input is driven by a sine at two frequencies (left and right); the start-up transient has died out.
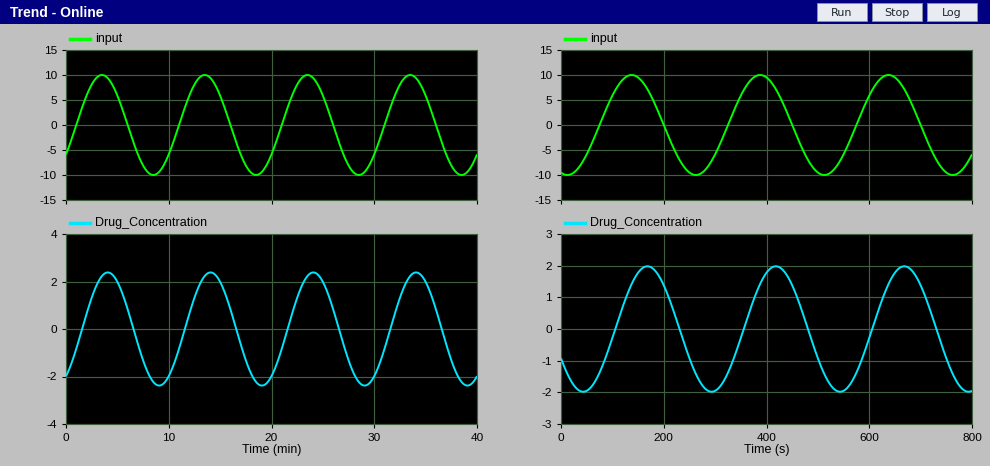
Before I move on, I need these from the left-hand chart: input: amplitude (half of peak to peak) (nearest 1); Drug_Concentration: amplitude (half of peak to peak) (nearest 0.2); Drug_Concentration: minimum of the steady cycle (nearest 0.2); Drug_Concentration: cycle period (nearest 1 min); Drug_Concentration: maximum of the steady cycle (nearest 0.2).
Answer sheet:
10
2.4
-2.4
10 min
2.4
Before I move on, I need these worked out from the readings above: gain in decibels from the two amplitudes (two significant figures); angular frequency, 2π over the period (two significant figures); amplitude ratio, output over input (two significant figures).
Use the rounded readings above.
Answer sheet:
-12 dB
0.63 rad/min
0.24
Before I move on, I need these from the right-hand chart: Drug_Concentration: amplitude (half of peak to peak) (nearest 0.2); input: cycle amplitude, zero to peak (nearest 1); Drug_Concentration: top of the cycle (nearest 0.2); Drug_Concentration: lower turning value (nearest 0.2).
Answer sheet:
2.0
10
2.0
-2.0
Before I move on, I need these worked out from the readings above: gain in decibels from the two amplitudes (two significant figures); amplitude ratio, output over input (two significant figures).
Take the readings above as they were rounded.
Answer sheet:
-14 dB
0.20
